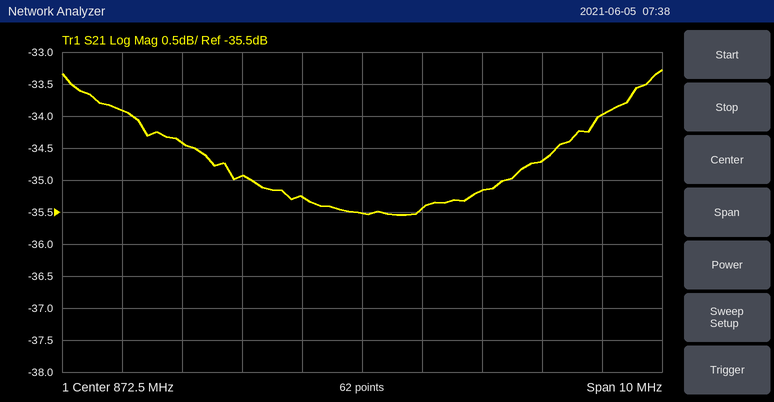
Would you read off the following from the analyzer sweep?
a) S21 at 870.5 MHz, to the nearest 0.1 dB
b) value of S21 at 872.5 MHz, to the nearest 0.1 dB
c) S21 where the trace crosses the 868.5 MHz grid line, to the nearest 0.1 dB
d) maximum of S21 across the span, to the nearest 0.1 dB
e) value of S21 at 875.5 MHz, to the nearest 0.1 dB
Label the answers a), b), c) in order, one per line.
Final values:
a) -34.9 dB
b) -35.5 dB
c) -33.9 dB
d) -33.3 dB
e) -34.7 dB
